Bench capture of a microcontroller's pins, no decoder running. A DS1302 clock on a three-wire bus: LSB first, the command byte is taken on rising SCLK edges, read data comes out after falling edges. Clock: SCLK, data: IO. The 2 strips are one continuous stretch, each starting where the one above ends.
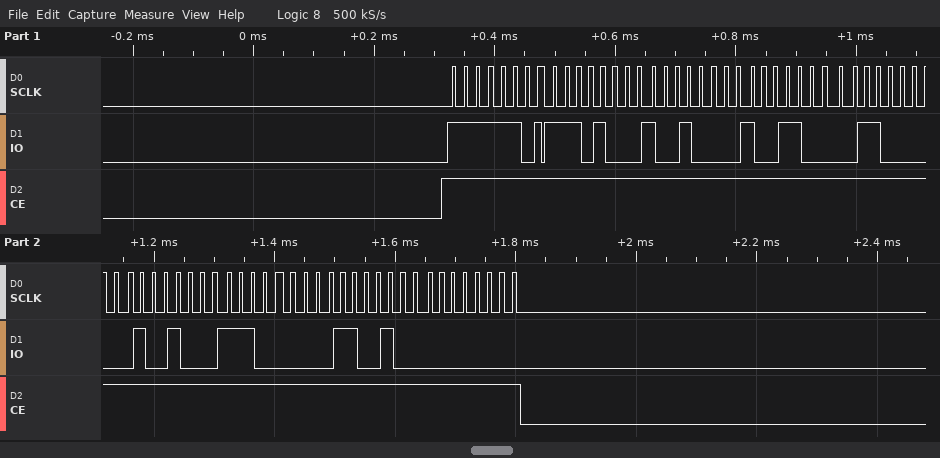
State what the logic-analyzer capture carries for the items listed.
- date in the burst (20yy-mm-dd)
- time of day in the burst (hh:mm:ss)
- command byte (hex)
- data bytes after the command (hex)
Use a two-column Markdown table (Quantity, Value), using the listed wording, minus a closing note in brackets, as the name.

| Quantity | Value |
|---|---|
| date in the burst | 2026-12-06 |
| time of day in the burst | 19:09:17 |
| command byte | 0xBF |
| data bytes after the command | 17 09 19 06 12 07 26 00 |
